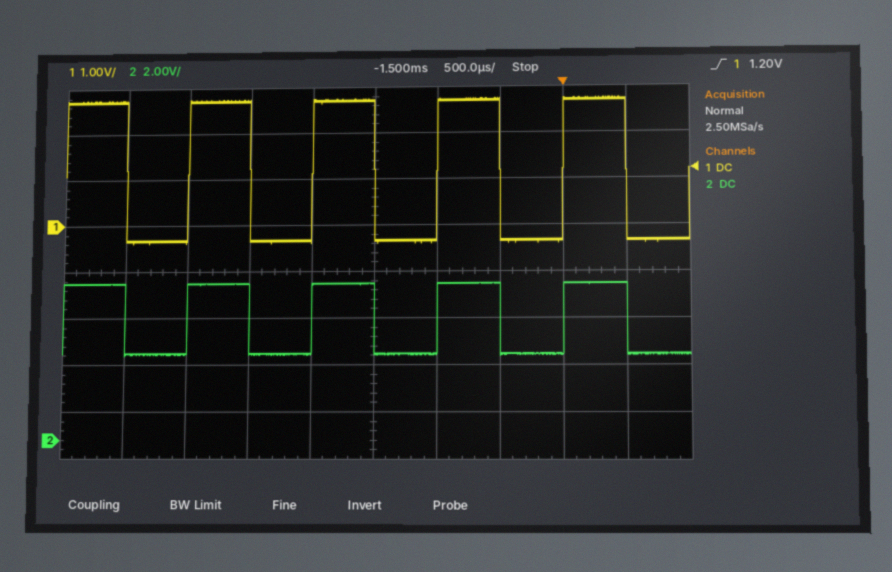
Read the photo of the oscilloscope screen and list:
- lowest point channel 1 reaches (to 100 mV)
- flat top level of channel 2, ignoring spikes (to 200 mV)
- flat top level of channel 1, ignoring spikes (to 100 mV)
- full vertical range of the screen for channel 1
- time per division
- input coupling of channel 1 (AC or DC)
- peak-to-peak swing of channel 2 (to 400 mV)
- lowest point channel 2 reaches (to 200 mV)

-400 mV
6.6 V
2.7 V
8 V
500 µs
DC
3.2 V
3.6 V
